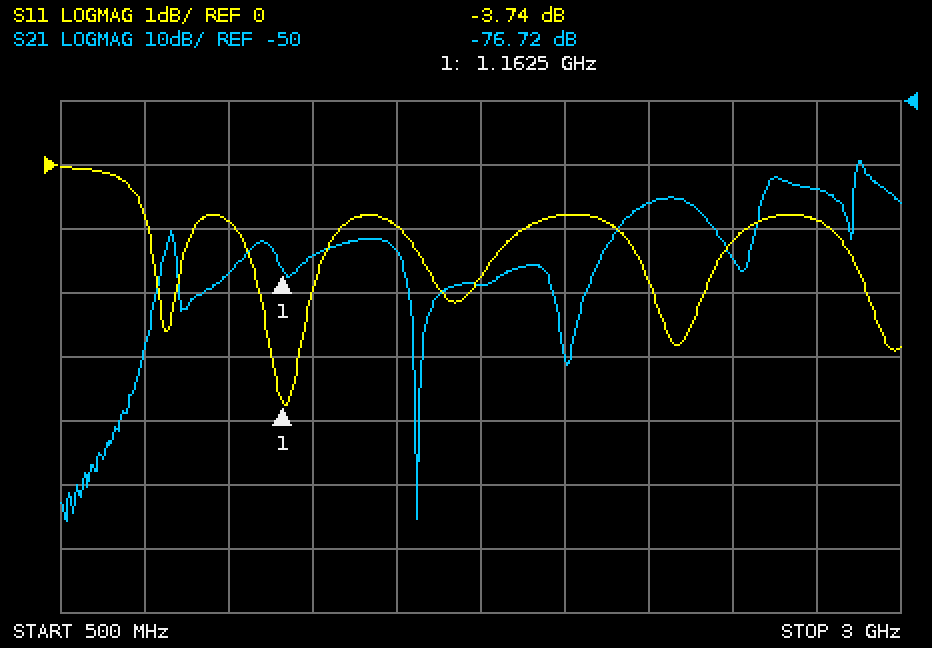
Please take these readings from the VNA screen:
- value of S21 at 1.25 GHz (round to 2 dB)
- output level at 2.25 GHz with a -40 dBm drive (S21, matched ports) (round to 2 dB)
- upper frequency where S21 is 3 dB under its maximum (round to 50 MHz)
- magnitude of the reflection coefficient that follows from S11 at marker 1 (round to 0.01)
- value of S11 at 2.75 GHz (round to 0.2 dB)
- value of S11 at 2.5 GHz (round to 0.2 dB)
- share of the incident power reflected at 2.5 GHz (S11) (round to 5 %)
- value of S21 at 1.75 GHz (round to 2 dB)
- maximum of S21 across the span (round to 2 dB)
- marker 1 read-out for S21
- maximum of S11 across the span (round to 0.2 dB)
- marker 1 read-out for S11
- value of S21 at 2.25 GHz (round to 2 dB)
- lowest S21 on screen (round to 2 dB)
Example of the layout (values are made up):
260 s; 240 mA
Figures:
-74 dB; -106 dBm; 2.90 GHz; 0.65; -0.8 dB; -1.2 dB; 75 %; -78 dB; -60 dB; -76.72 dB; 0.0 dB; -3.74 dB; -66 dB; -116 dB
